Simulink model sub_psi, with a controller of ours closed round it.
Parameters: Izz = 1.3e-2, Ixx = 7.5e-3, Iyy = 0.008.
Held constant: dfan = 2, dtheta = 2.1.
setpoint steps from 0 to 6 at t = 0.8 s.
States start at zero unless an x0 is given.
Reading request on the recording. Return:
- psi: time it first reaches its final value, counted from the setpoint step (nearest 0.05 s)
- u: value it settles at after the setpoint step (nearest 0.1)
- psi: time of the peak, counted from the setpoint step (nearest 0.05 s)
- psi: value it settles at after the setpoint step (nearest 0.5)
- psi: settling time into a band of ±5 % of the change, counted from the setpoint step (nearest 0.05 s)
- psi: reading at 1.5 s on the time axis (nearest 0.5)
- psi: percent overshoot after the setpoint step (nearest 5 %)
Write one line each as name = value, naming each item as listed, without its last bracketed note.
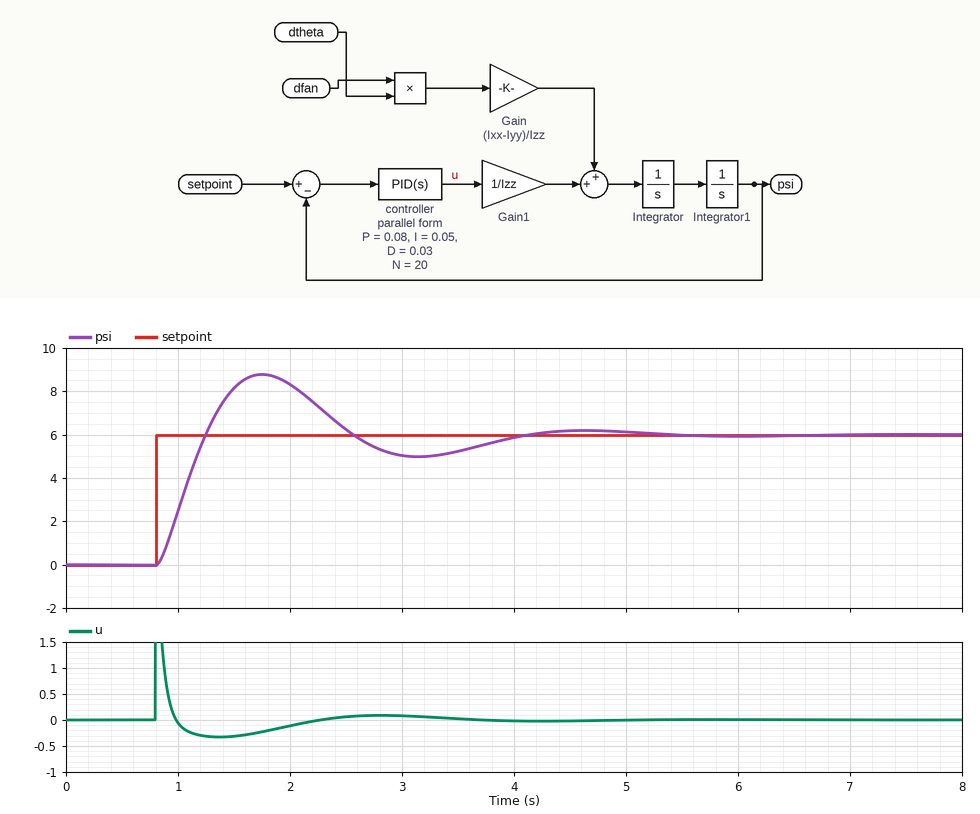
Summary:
psi: time it first reaches its final value, counted from the setpoint step = 0.45 s
u: value it settles at after the setpoint step = 0.0
psi: time of the peak, counted from the setpoint step = 0.95 s
psi: value it settles at after the setpoint step = 6.0
psi: settling time into a band of ±5 % of the change, counted from the setpoint step = 3.05 s
psi: reading at 1.5 s on the time axis = 8.0
psi: percent overshoot after the setpoint step = 45 %
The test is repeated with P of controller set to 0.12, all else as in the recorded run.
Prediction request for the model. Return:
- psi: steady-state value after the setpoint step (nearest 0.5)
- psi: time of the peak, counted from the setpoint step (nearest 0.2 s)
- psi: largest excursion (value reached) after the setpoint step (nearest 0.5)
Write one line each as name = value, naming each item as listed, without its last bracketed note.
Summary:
psi: steady-state value after the setpoint step = 6.0
psi: time of the peak, counted from the setpoint step = 0.8 s
psi: largest excursion (value reached) after the setpoint step = 9.0
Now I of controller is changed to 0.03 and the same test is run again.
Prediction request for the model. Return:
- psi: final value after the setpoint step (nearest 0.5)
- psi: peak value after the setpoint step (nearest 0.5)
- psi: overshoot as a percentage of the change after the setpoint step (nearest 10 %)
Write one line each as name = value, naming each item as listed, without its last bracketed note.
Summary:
psi: final value after the setpoint step = 6.0
psi: peak value after the setpoint step = 8.5
psi: overshoot as a percentage of the change after the setpoint step = 40 %
